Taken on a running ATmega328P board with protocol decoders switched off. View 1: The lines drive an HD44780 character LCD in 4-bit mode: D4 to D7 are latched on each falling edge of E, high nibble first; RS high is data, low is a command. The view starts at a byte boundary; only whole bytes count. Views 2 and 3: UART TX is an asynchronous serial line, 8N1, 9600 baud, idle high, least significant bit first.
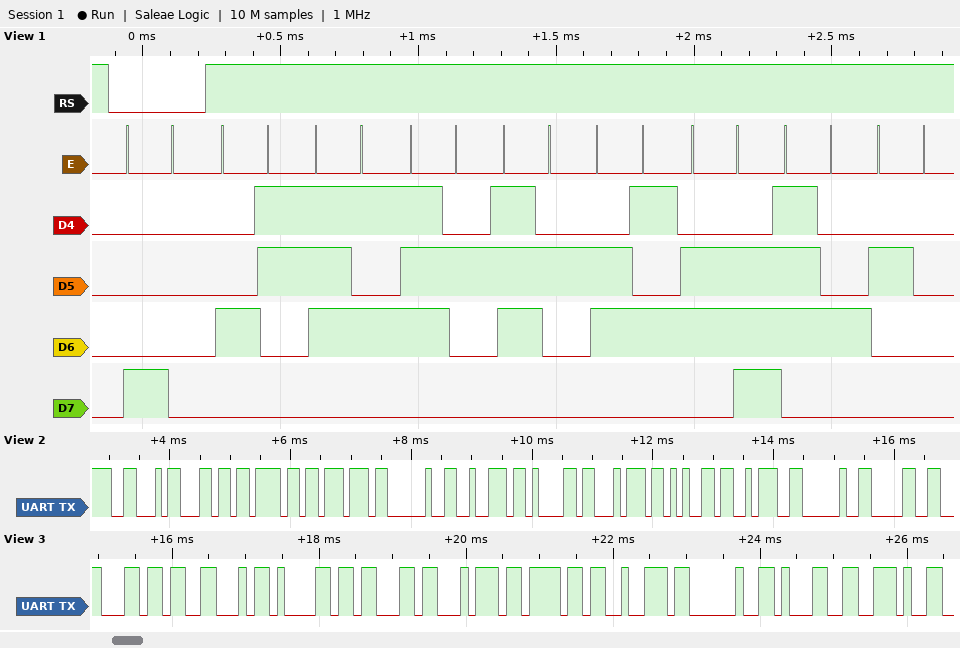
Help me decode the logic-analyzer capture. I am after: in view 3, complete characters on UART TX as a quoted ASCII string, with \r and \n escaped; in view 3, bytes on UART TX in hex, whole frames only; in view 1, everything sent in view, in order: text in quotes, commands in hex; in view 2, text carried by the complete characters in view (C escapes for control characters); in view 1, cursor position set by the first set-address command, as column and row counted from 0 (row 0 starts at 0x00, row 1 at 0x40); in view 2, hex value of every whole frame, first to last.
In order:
"lFactor 1."
6C 46 61 63 74 6F 72 20 31 2E
0x80 "Current "
"Flow rate: 0"
column 0, row 0
46 6C 6F 77 20 72 61 74 65 3A 20 30
